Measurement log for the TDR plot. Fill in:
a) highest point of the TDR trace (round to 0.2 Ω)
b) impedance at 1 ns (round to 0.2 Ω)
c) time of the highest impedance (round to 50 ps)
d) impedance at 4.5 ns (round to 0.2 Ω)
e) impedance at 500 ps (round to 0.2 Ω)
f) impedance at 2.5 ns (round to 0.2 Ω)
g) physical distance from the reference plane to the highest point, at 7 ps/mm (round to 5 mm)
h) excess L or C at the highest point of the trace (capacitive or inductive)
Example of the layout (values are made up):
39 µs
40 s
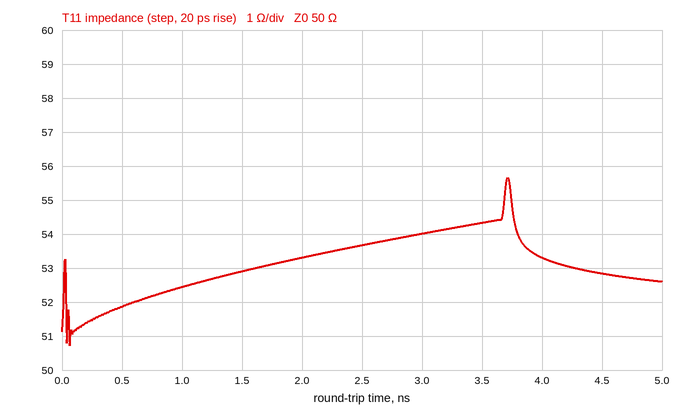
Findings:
55.6 Ω
52.4 Ω
3.70 ns
52.8 Ω
51.8 Ω
53.6 Ω
265 mm
inductive
